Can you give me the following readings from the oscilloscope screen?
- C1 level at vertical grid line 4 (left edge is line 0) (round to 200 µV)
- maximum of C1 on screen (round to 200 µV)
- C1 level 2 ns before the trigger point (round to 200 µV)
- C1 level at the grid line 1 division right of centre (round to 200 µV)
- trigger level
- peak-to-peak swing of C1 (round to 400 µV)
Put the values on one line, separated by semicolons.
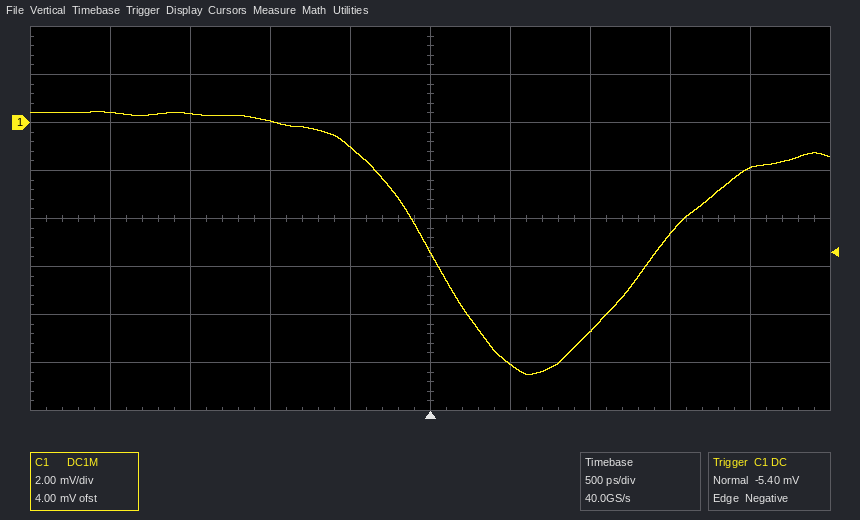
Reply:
-1.0 mV; 400 µV; 400 µV; -10.0 mV; -5.40 mV; 10.8 mV
